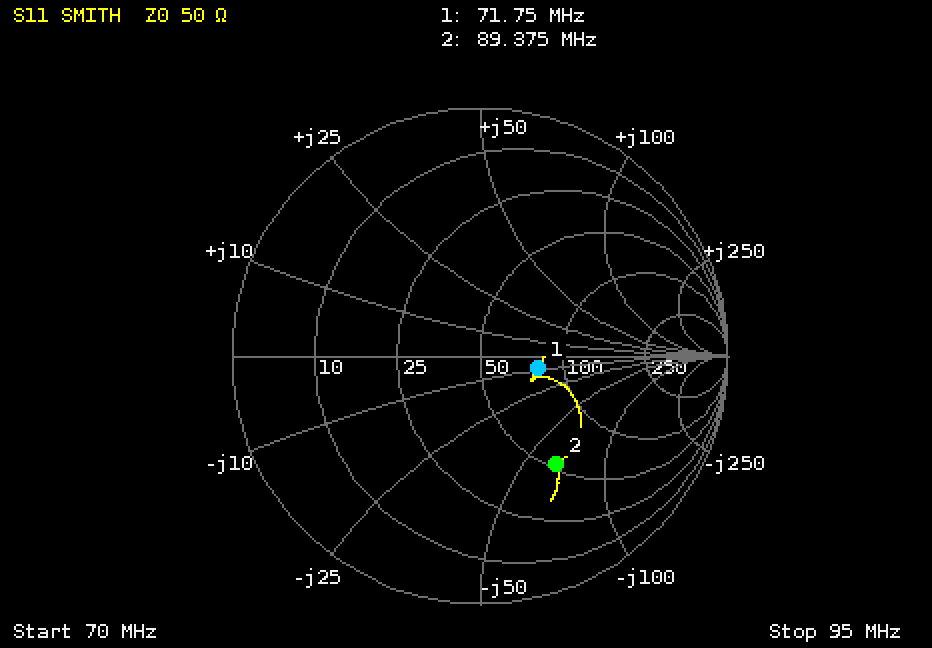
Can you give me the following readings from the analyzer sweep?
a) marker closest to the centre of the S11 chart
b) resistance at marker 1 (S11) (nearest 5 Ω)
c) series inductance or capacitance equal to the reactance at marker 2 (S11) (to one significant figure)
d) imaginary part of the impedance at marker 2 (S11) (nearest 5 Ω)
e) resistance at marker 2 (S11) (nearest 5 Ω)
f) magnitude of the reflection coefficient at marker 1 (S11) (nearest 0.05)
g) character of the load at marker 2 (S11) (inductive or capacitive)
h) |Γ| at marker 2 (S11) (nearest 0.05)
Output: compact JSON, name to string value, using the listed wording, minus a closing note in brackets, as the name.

{"marker closest to the centre of the S11 chart": "marker 1", "resistance at marker 1 (S11)": "80 Ω", "series inductance or capacitance equal to the reactance at marker 2 (S11)": "30 pF", "imaginary part of the impedance at marker 2 (S11)": "-65 Ω", "resistance at marker 2 (S11)": "55 Ω", "magnitude of the reflection coefficient at marker 1 (S11)": "0.25", "character of the load at marker 2 (S11)": "capacitive", "|Γ| at marker 2 (S11)": "0.55"}
